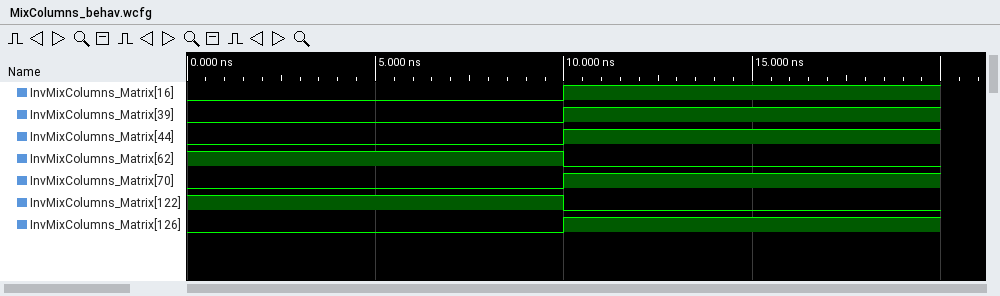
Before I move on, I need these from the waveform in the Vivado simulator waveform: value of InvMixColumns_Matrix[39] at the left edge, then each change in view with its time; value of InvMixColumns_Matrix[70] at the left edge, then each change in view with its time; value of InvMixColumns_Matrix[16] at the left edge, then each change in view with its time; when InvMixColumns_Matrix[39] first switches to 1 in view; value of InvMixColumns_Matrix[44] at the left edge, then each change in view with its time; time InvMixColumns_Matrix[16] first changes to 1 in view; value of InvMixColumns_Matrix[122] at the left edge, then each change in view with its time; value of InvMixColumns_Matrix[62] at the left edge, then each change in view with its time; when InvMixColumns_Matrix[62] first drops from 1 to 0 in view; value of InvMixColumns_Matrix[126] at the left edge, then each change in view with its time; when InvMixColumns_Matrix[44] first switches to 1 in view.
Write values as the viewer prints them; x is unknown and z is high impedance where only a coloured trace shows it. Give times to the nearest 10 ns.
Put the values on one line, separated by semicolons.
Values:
0, 1 at 10 ns; 0, 1 at 10 ns; 0, 1 at 10 ns; 10 ns; 0, 1 at 10 ns; 10 ns; 1, 0 at 10 ns; 1, 0 at 10 ns; 10 ns; 0, 1 at 10 ns; 10 ns
